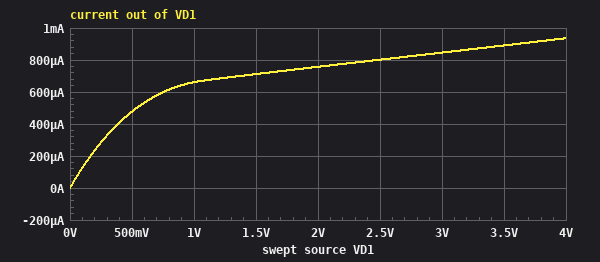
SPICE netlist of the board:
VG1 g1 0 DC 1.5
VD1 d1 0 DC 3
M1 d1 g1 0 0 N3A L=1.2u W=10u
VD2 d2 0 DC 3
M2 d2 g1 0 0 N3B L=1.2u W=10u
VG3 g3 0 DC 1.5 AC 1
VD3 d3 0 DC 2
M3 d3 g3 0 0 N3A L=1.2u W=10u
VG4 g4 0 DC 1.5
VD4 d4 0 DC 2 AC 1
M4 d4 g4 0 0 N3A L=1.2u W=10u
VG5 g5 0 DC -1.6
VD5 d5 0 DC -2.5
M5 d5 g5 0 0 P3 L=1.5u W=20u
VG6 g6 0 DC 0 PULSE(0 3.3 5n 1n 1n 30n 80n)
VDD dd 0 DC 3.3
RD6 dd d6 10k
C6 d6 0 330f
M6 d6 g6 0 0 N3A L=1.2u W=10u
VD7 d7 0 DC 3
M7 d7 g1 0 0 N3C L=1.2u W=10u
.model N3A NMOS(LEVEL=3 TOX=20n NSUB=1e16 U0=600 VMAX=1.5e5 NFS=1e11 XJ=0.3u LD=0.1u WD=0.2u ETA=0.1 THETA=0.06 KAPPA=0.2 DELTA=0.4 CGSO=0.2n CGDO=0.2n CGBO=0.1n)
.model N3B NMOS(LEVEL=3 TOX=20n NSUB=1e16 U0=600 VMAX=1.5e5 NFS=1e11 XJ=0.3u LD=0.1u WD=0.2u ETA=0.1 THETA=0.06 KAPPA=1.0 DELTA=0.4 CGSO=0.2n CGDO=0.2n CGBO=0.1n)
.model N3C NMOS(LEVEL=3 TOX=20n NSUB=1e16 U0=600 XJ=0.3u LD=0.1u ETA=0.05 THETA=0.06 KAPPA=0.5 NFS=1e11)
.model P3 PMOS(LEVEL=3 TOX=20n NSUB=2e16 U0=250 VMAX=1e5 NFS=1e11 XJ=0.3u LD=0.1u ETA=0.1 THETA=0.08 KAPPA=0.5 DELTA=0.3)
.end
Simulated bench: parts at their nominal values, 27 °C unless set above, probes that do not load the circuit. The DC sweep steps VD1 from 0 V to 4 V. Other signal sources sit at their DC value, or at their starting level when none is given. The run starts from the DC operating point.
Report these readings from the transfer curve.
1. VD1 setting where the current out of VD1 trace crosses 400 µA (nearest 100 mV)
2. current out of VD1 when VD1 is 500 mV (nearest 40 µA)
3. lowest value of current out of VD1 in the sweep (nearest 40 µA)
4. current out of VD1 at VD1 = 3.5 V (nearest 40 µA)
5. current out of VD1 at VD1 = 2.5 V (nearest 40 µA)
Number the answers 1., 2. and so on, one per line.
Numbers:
1. 400 mV
2. 480 µA
3. 0 A
4. 880 µA
5. 800 µA
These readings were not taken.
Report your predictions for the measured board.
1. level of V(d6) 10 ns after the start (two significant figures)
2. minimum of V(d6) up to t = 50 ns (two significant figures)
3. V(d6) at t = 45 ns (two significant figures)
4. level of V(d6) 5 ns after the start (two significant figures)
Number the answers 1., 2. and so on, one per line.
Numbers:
1. 120 mV
2. 120 mV
3. 3.0 V
4. 3.2 V
